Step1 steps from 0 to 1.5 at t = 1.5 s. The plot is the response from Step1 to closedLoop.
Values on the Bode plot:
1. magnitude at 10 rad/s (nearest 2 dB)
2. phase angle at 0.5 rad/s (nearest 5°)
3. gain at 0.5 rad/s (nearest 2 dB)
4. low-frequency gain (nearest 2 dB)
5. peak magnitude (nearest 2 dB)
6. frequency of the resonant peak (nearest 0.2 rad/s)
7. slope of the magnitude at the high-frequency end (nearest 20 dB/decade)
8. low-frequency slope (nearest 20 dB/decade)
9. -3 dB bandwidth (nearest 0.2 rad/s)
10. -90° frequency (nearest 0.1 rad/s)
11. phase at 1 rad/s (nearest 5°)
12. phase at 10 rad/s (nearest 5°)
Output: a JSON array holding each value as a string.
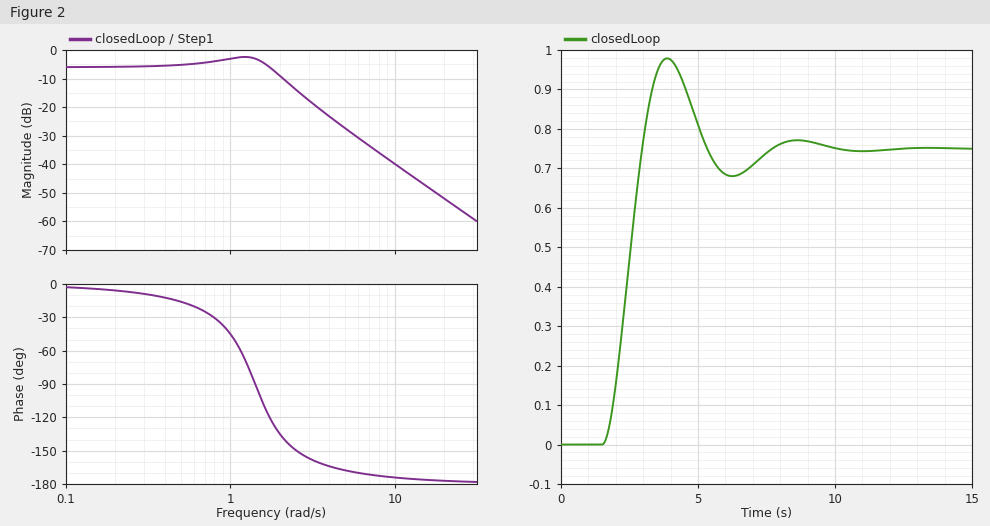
["-40 dB", "-15°", "-6 dB", "-6 dB", "-2 dB", "1.2 rad/s", "-40 dB/decade", "0 dB/decade", "2.0 rad/s", "1.4 rad/s", "-45°", "-175°"]
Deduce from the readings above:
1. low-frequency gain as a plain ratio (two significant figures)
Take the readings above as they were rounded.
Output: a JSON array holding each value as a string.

["0.50"]
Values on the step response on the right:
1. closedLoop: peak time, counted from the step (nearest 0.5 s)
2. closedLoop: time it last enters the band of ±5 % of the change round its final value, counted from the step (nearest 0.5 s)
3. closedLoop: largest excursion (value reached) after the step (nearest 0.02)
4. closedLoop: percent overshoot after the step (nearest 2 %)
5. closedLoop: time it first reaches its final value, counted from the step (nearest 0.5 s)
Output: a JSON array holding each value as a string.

["2.5 s", "5.5 s", "0.98", "30 %", "1.5 s"]
